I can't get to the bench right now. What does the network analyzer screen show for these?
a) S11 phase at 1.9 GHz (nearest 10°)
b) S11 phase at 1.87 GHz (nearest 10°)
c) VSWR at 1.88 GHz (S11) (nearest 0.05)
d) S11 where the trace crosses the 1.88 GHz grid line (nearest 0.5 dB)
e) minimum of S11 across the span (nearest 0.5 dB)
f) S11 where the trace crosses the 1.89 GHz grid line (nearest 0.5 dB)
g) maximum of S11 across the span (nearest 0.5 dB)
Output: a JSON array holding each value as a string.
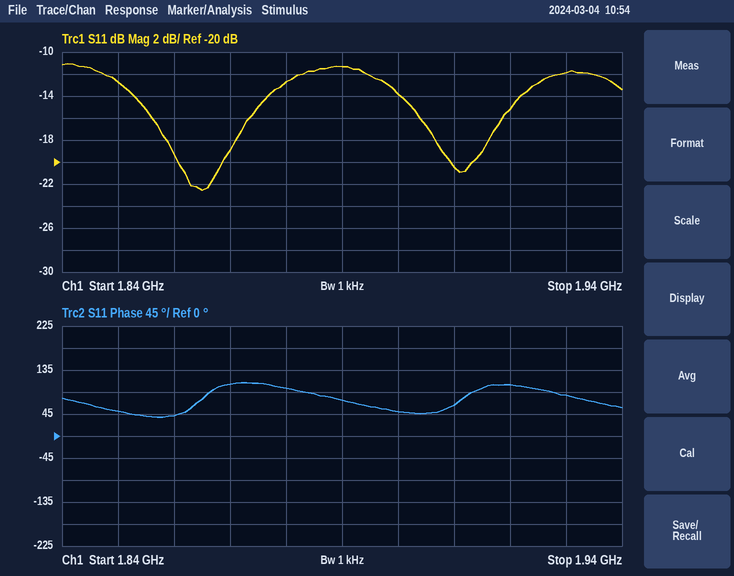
["50°", "110°", "1.60", "-12.5 dB", "-22.5 dB", "-11.5 dB", "-11.0 dB"]
